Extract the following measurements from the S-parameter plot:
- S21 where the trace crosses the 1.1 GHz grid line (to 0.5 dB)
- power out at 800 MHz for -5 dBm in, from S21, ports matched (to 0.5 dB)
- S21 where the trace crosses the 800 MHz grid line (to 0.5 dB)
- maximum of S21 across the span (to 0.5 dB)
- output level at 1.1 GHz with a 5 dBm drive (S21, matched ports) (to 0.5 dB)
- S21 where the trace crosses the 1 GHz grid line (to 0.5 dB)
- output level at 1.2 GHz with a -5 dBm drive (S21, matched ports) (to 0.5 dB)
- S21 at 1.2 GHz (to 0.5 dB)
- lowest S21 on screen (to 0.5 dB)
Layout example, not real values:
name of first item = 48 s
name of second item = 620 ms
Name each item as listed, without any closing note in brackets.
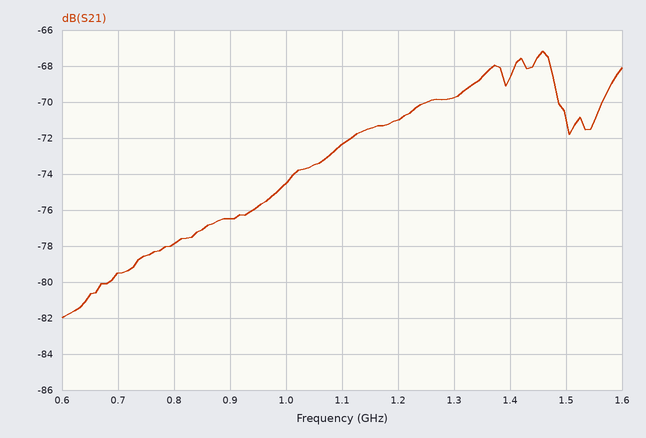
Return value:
S21 where the trace crosses the 1.1 GHz grid line = -72.5 dB
power out at 800 MHz for -5 dBm in, from S21, ports matched = -83.0 dBm
S21 where the trace crosses the 800 MHz grid line = -78.0 dB
maximum of S21 across the span = -67.0 dB
output level at 1.1 GHz with a 5 dBm drive (S21, matched ports) = -67.5 dBm
S21 where the trace crosses the 1 GHz grid line = -74.5 dB
output level at 1.2 GHz with a -5 dBm drive (S21, matched ports) = -76.0 dBm
S21 at 1.2 GHz = -71.0 dB
lowest S21 on screen = -82.0 dB
